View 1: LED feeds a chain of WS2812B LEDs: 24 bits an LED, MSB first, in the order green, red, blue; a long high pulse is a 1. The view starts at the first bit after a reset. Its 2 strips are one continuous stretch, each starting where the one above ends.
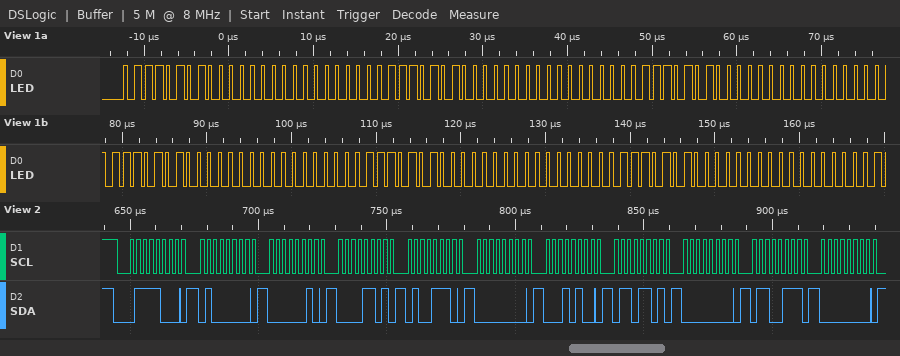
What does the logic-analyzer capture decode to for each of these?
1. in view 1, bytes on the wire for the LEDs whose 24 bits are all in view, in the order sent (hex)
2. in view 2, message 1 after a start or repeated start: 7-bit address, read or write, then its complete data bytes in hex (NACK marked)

75 00 00 75 00 00 75 00 00 75 00 00 75 00 00 75 00 00
0x3C write: 40 02 0D 4E 00 14 6D 00 67 00
